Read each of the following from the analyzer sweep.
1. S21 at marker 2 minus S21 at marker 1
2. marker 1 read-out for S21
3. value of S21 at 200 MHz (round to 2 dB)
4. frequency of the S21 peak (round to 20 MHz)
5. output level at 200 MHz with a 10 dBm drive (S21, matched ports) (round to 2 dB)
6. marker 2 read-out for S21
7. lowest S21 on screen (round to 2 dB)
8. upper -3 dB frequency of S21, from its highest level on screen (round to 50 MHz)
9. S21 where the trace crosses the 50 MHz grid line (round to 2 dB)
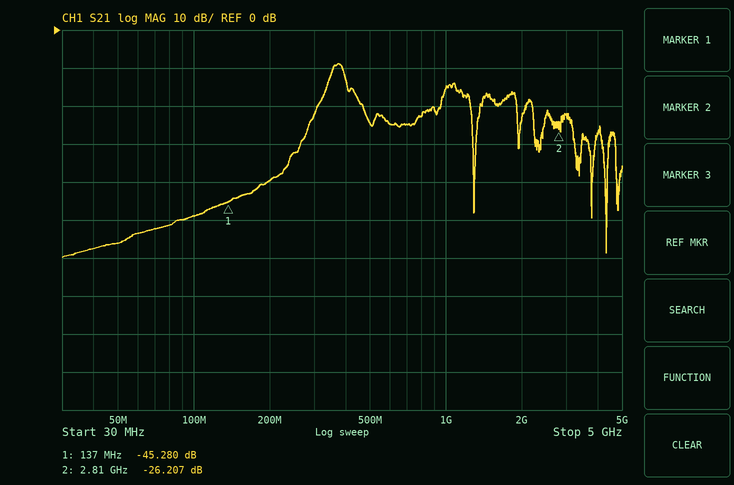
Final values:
19.073 dB
-45.280 dB
-40 dB
380 MHz
-30 dBm
-26.207 dB
-60 dB
400 MHz
-56 dB
